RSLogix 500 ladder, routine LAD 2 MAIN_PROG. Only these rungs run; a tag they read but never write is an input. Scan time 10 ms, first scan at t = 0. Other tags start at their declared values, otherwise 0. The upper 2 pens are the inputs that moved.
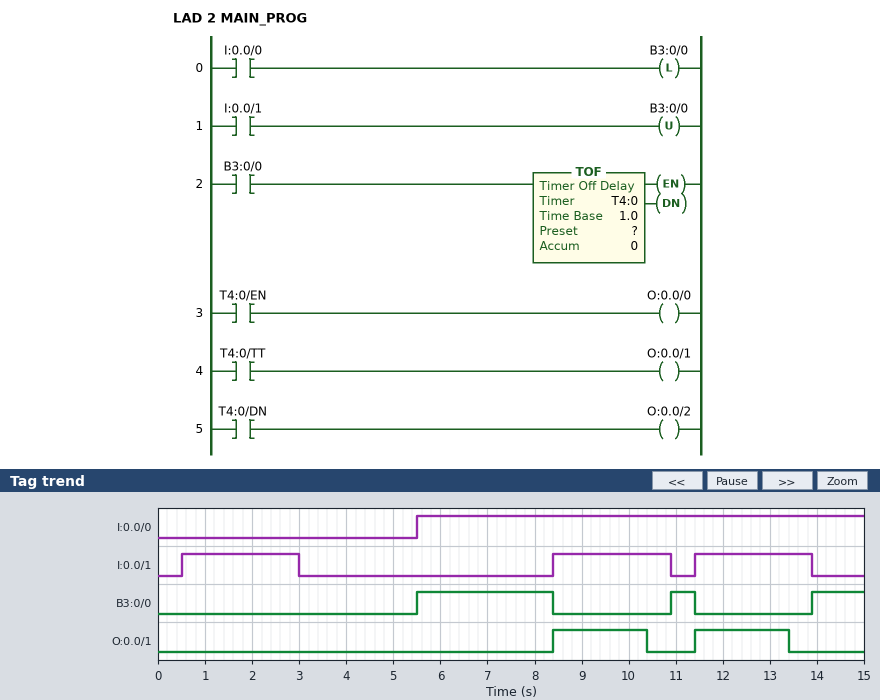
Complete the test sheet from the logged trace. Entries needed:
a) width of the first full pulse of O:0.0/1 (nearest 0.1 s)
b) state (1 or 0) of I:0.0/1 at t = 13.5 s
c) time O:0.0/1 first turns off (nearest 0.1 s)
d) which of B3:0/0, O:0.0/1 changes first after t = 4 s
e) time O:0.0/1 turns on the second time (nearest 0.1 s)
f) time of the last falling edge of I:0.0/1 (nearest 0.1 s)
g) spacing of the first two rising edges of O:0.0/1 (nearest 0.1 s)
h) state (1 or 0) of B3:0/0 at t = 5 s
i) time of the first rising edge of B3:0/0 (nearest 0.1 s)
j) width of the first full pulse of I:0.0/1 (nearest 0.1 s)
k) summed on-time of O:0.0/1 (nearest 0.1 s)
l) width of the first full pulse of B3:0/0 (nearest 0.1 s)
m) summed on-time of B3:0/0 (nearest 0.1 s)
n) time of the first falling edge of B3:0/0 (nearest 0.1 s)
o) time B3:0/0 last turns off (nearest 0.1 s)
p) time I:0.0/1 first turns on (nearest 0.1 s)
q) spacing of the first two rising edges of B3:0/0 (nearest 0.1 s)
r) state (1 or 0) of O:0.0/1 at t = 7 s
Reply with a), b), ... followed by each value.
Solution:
a) 2.0 s
b) 1
c) 10.4 s
d) B3:0/0
e) 11.4 s
f) 13.9 s
g) 3.0 s
h) 0
i) 5.5 s
j) 2.5 s
k) 4.0 s
l) 2.9 s
m) 4.5 s
n) 8.4 s
o) 11.4 s
p) 0.5 s
q) 5.4 s
r) 0
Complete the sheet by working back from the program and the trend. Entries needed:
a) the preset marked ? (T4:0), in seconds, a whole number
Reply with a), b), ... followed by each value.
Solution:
a) 2 s
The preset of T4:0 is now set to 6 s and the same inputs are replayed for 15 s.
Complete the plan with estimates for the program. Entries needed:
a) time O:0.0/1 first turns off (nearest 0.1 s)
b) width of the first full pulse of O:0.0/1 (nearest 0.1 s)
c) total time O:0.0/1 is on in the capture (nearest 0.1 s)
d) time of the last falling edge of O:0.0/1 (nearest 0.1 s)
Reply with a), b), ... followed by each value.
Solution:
a) 10.9 s
b) 2.5 s
c) 5.0 s
d) 13.9 s
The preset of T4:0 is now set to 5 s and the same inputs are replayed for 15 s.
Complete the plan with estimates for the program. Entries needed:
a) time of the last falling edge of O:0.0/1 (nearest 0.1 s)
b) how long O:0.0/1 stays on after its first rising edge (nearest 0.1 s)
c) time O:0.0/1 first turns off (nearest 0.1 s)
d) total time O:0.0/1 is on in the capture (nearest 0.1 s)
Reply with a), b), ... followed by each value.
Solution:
a) 13.9 s
b) 2.5 s
c) 10.9 s
d) 5.0 s
